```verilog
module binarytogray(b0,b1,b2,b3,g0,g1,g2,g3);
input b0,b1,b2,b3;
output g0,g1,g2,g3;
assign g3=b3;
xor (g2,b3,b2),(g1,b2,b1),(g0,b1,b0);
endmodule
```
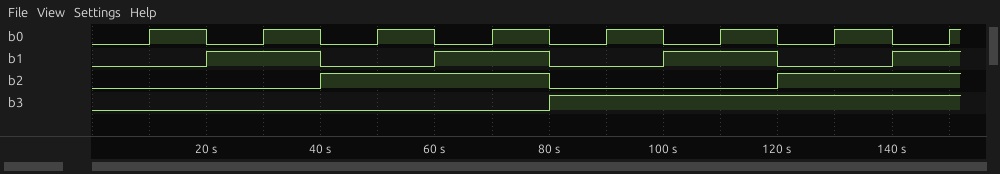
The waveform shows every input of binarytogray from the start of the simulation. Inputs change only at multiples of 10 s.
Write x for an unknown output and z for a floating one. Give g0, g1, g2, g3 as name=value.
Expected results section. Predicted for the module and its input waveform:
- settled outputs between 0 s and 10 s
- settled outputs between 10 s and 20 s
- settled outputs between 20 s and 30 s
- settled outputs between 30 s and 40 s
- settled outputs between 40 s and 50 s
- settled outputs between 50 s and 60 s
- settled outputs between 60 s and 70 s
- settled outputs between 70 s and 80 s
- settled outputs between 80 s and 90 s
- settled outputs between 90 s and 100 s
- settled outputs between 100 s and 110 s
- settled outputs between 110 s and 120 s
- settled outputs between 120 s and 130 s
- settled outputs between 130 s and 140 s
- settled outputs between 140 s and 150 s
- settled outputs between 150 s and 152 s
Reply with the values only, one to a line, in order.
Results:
g0=0, g1=0, g2=0, g3=0
g0=1, g1=0, g2=0, g3=0
g0=1, g1=1, g2=0, g3=0
g0=0, g1=1, g2=0, g3=0
g0=0, g1=1, g2=1, g3=0
g0=1, g1=1, g2=1, g3=0
g0=1, g1=0, g2=1, g3=0
g0=0, g1=0, g2=1, g3=0
g0=0, g1=0, g2=1, g3=1
g0=1, g1=0, g2=1, g3=1
g0=1, g1=1, g2=1, g3=1
g0=0, g1=1, g2=1, g3=1
g0=0, g1=1, g2=0, g3=1
g0=1, g1=1, g2=0, g3=1
g0=1, g1=0, g2=0, g3=1
g0=0, g1=0, g2=0, g3=1
